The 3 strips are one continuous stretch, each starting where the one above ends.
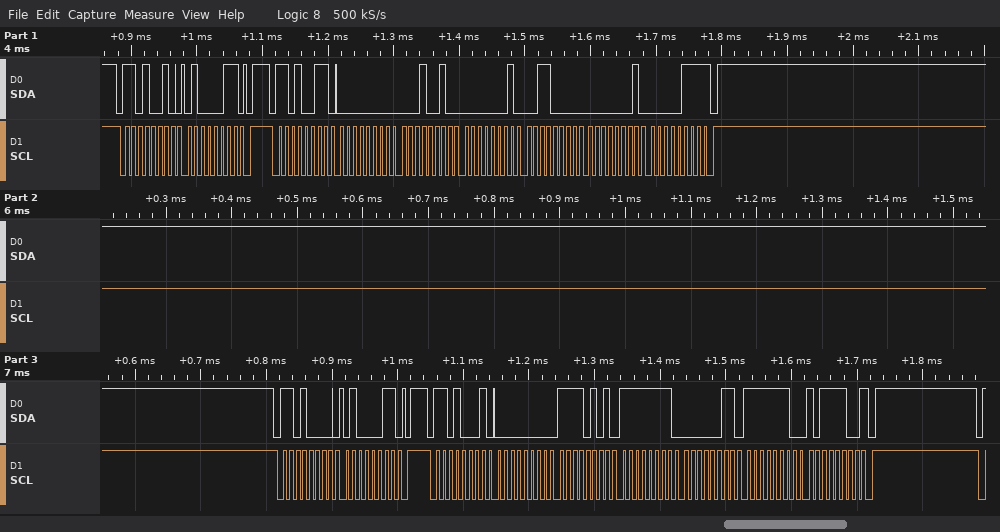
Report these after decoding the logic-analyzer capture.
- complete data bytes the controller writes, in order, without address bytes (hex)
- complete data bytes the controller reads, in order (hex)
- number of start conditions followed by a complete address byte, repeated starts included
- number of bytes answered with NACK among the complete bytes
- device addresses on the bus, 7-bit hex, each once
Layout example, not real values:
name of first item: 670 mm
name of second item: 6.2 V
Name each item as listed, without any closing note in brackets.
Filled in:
complete data bytes the controller writes, in order, without address bytes: 43 43
complete data bytes the controller reads, in order: 00 12 01 30 01 07 00 F5 FF 03 FE BC
number of start conditions followed by a complete address byte, repeated starts included: 4
number of bytes answered with NACK among the complete bytes: 2
device addresses on the bus, 7-bit hex, each once: 0x69 0x68
